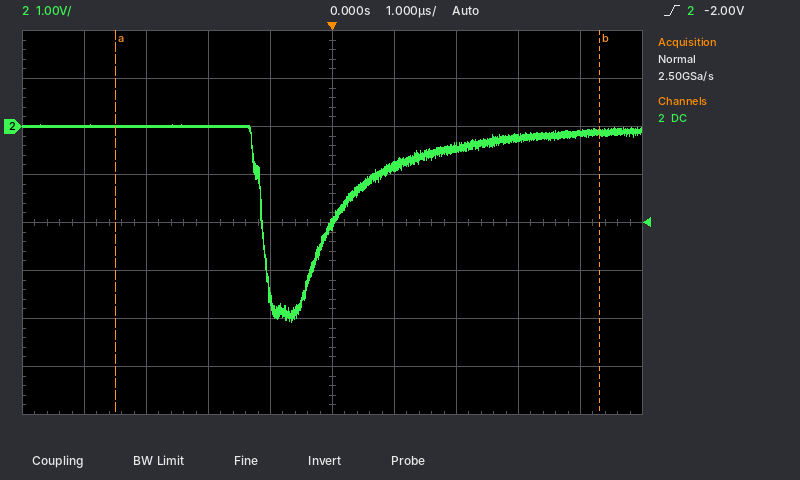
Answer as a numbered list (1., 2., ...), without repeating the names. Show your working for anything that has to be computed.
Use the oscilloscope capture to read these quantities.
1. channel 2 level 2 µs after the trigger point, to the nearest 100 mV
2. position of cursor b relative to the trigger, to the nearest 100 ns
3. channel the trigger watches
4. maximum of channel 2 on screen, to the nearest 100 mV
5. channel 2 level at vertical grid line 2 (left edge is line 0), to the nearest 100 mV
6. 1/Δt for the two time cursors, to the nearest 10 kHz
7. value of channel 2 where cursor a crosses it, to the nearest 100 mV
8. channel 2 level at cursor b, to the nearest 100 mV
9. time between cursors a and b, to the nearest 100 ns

1. -400 mV
2. +4.3 µs
3. channel 2
4. 0.0 V
5. 0.0 V
6. 1 / 7.8 µs ≈ 130 kHz
7. 0.0 V
8. -100 mV
9. 7.8 µs
